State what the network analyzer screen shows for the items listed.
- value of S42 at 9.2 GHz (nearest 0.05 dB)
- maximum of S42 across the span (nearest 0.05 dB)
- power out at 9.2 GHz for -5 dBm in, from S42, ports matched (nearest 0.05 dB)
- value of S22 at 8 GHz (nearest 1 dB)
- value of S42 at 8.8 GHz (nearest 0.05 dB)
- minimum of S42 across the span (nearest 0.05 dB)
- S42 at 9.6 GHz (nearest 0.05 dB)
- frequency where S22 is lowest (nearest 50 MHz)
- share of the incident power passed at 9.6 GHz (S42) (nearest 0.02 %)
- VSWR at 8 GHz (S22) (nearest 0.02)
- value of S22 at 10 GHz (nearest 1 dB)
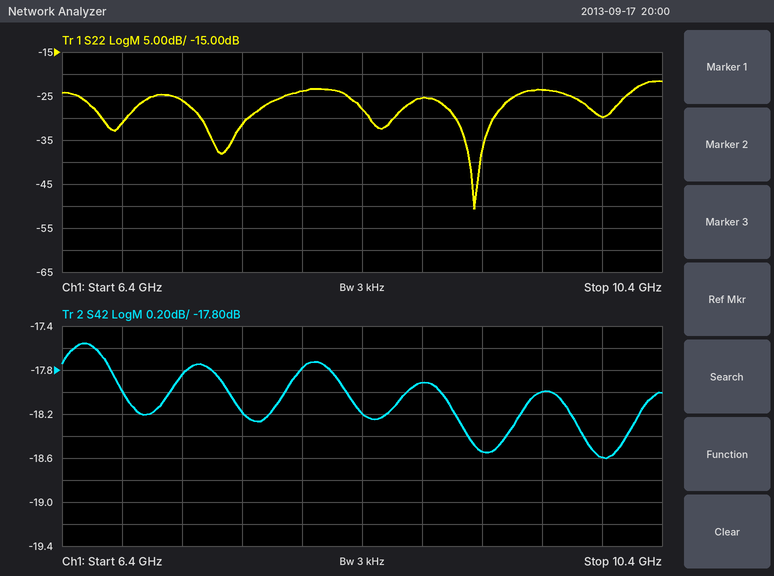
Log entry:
-18.55 dB
-17.55 dB
-23.55 dBm
-24 dB
-17.90 dB
-18.60 dB
-18.00 dB
9.15 GHz
1.58 %
1.14
-30 dB
